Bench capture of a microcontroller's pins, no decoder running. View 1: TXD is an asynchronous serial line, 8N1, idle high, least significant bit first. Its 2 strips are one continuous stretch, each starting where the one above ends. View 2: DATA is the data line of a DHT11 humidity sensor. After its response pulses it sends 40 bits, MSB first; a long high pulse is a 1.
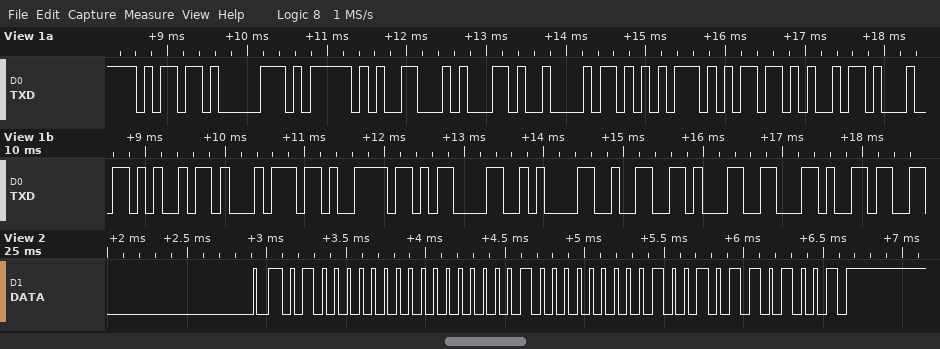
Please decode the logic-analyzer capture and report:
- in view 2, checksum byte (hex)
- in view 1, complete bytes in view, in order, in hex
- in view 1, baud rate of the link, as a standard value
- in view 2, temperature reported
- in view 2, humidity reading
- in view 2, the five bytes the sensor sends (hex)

0x69
0x6D 0x70 0x5F 0x46 0x2C 0x68 0x75 0x6D 0x69 0x64 0x69 0x74 0x79 0x0D 0x0A 0x32 0x31 0x2C
9600 baud
32.9 °C
64 %
40 00 20 09 69
